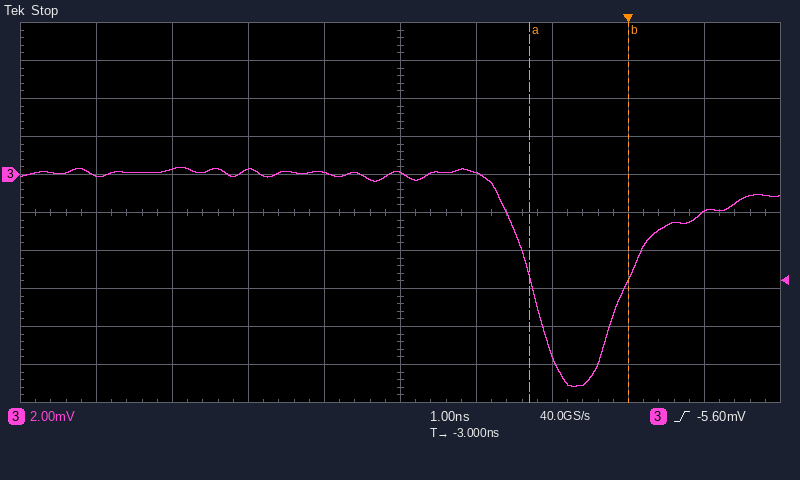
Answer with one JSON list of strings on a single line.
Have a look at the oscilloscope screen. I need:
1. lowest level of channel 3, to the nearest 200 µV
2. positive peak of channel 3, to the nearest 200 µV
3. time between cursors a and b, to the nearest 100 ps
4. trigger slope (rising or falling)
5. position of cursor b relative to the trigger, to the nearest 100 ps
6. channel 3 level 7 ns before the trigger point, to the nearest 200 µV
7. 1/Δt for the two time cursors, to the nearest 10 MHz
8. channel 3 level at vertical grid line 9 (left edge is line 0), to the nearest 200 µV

["-11.2 mV", "400 µV", "1.3 ns", "rising", "0.0 ns", "0.0 mV", "770 MHz", "-2.0 mV"]
